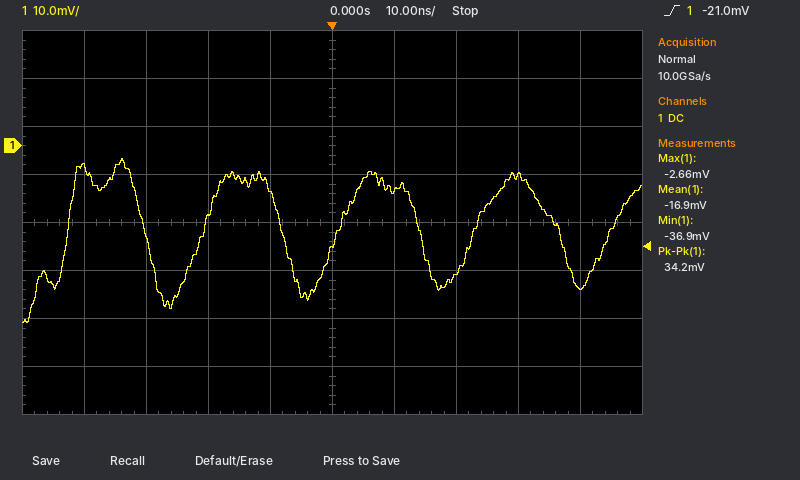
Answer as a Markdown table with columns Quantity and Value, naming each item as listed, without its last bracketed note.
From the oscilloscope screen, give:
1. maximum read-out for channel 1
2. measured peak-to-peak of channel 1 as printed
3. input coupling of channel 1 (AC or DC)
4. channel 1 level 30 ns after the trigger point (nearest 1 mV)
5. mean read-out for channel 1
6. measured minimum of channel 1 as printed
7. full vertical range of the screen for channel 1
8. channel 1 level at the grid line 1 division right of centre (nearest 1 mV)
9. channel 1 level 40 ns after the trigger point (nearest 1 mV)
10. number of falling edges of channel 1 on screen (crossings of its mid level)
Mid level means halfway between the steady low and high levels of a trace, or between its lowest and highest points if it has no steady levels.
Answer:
| Quantity | Value |
|---|---|
| maximum read-out for channel 1 | -2.66 mV |
| measured peak-to-peak of channel 1 as printed | 34.2 mV |
| input coupling of channel 1 | DC |
| channel 1 level 30 ns after the trigger point | -6 mV |
| mean read-out for channel 1 | -16.9 mV |
| measured minimum of channel 1 as printed | -36.9 mV |
| full vertical range of the screen for channel 1 | 80 mV |
| channel 1 level at the grid line 1 division right of centre | -9 mV |
| channel 1 level 40 ns after the trigger point | -30 mV |
| number of falling edges of channel 1 on screen | 4 |
